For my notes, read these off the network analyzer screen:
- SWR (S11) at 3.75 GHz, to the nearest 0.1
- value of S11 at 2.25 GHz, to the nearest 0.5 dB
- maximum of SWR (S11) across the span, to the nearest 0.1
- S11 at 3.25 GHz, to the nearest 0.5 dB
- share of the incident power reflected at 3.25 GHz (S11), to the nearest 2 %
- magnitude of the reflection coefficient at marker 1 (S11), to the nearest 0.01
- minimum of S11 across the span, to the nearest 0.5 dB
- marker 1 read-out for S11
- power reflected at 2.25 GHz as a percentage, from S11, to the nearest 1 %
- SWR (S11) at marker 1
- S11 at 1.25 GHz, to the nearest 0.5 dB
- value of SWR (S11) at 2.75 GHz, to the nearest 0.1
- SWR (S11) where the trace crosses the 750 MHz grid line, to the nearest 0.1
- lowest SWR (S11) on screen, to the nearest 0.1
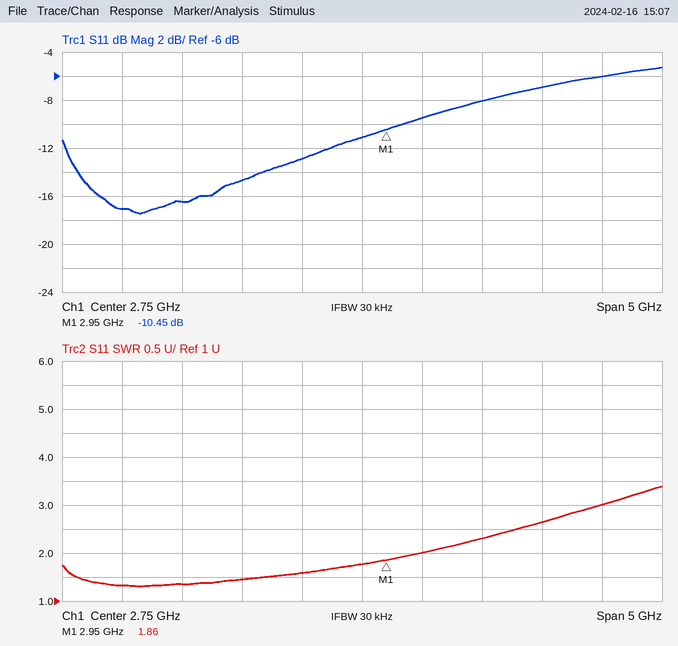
2.3
-13.0 dB
3.4
-9.5 dB
12 %
0.30
-17.5 dB
-10.45 dB
5 %
1.86
-16.5 dB
1.8
1.3
1.3
